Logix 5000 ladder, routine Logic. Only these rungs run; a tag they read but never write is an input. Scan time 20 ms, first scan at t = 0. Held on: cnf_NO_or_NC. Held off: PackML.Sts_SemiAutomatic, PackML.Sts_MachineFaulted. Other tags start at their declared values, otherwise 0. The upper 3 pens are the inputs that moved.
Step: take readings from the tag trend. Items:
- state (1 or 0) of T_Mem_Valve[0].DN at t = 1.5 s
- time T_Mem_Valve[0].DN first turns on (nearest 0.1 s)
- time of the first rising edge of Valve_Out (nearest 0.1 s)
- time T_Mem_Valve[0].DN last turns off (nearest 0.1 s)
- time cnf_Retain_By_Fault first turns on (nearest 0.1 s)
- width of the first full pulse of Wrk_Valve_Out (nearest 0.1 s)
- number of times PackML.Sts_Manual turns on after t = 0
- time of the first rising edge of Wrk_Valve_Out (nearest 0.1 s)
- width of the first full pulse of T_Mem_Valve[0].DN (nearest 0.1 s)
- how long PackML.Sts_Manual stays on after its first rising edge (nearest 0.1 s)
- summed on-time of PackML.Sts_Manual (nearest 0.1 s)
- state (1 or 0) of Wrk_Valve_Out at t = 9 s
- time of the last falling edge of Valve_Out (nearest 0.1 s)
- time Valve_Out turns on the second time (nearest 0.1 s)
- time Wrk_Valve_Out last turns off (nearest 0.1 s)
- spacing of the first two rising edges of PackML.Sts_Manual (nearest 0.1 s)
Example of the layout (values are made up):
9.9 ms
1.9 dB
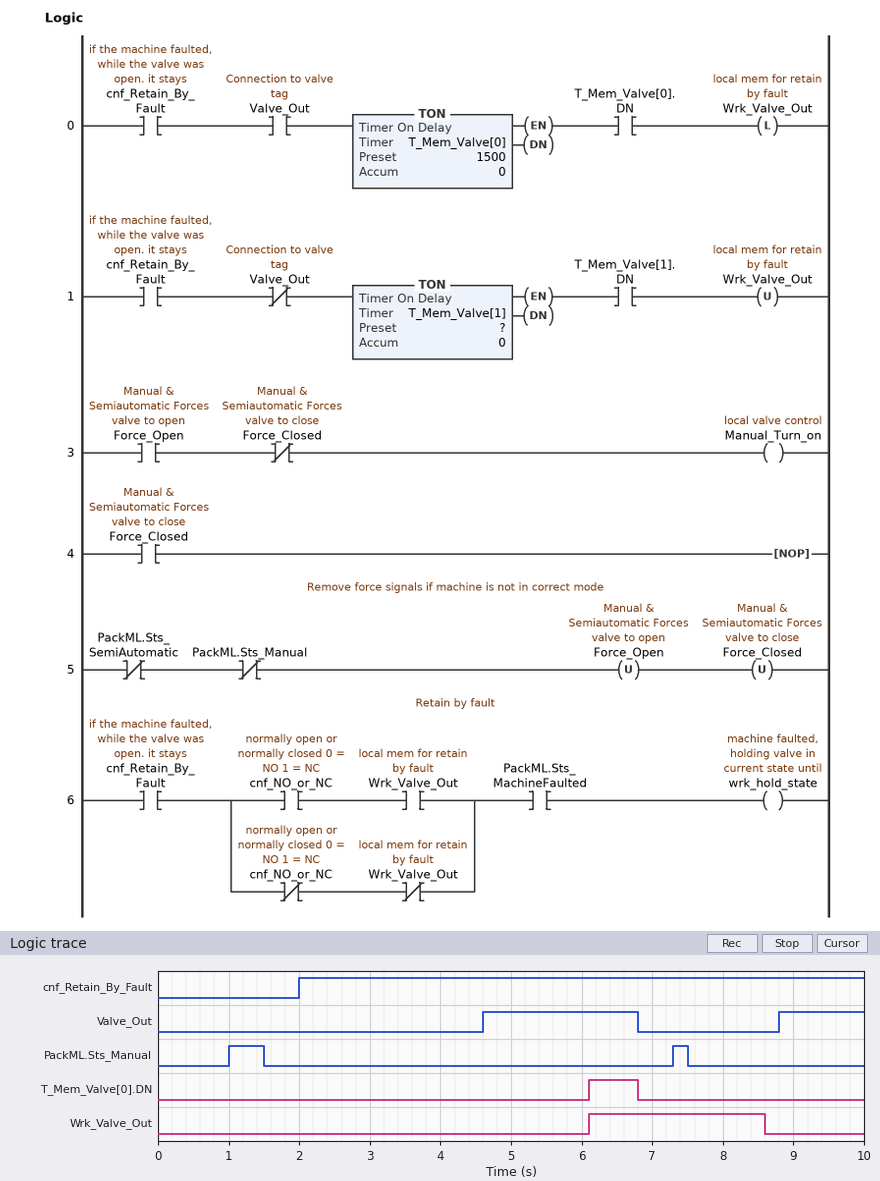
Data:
0
6.1 s
4.6 s
6.8 s
2.0 s
2.5 s
2
6.1 s
0.7 s
0.5 s
0.7 s
0
6.8 s
8.8 s
8.6 s
6.3 s
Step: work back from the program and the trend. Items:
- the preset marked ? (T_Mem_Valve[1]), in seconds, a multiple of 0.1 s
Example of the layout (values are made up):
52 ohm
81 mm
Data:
1.8 s
